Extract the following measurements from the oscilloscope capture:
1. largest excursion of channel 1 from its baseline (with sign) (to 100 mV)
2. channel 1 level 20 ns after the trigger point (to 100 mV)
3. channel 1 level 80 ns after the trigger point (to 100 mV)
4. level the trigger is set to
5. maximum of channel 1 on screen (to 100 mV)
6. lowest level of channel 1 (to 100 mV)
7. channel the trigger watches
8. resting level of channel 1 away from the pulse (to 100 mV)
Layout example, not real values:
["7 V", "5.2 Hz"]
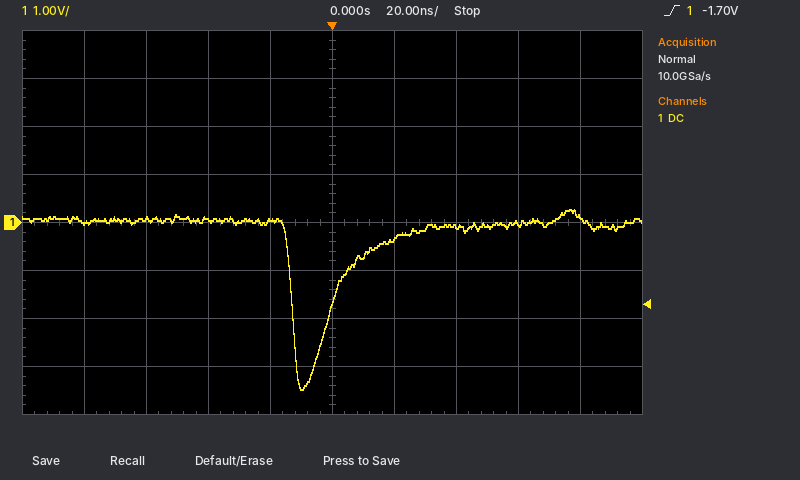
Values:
["-3.5 V", "-300 mV", "100 mV", "-1.70 V", "300 mV", "-3.5 V", "channel 1", "0.0 V"]
